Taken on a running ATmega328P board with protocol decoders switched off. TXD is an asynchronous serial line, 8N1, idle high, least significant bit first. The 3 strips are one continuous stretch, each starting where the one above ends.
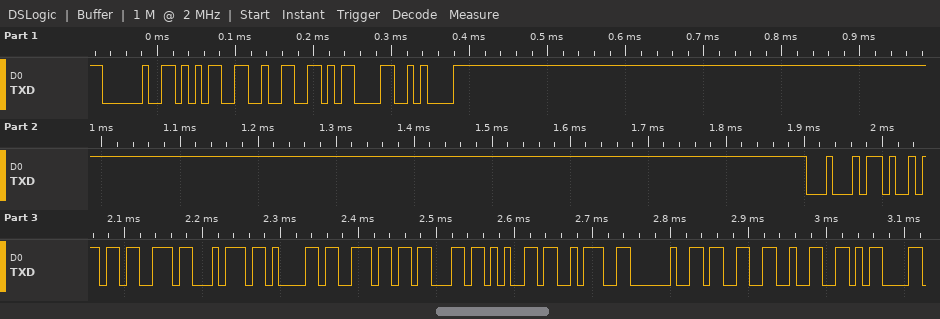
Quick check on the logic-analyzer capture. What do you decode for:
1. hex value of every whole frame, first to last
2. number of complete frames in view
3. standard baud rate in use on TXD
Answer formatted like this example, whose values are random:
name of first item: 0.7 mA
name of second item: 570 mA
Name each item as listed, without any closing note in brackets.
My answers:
hex value of every whole frame, first to last: 0x20 0x35 0x32 0x0D 0x0A 0x44 0x69 0x73 0x74 0x61 0x6E 0x63 0x65 0x3A 0x20 0x33 0x32 0x0D
number of complete frames in view: 18
standard baud rate in use on TXD: 115200 baud
